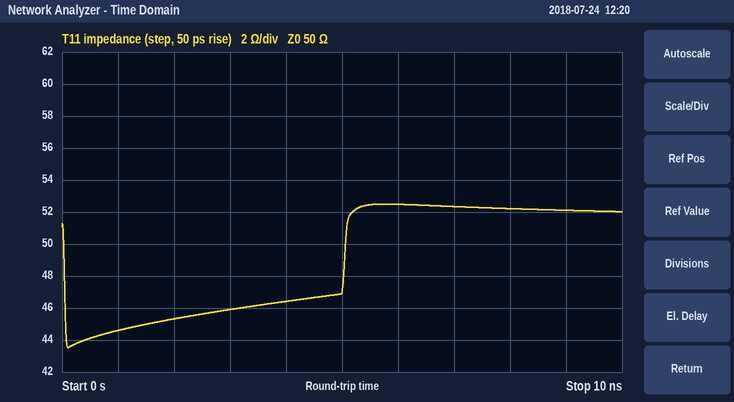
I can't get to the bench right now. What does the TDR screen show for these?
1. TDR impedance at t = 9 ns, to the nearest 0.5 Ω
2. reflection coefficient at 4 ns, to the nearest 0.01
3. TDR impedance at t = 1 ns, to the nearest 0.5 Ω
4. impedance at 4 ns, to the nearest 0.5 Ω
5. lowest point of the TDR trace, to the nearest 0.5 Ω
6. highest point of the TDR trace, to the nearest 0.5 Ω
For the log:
52.0 Ω
-0.04
44.5 Ω
46.5 Ω
43.5 Ω
52.5 Ω
